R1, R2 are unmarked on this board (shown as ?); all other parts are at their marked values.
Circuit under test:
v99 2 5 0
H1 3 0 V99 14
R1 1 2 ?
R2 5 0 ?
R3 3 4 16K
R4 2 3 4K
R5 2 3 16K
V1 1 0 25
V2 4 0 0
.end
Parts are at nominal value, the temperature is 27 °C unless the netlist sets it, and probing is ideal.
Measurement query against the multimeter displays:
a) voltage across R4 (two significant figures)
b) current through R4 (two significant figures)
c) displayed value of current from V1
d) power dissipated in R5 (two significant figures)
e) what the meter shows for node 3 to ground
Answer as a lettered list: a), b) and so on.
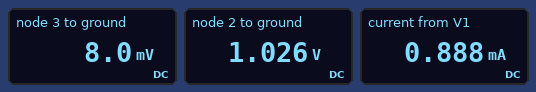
a) 1.0 V
b) 250 µA
c) 0.888 mA
d) 65 µW
e) 8.0 mV
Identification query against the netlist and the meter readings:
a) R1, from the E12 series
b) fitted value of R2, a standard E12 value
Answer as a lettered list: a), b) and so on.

a) 27 kΩ
b) 1.8 kΩ
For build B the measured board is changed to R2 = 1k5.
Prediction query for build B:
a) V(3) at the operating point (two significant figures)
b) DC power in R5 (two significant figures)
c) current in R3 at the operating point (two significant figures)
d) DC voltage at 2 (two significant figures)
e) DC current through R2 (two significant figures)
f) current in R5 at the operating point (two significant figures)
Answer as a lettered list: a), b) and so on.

a) 8.5 mV
b) 51 µW
c) 530 nA
d) 910 mV
e) 610 µA
f) 57 µA
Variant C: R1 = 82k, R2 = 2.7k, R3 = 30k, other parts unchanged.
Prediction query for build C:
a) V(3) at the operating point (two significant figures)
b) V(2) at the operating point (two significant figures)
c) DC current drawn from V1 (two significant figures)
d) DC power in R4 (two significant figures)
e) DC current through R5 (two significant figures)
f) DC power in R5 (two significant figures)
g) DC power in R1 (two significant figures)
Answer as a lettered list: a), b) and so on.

a) 2.3 mV
b) 440 mV
c) 300 µA
d) 48 µW
e) 27 µA
f) 12 µW
g) 7.4 mW
